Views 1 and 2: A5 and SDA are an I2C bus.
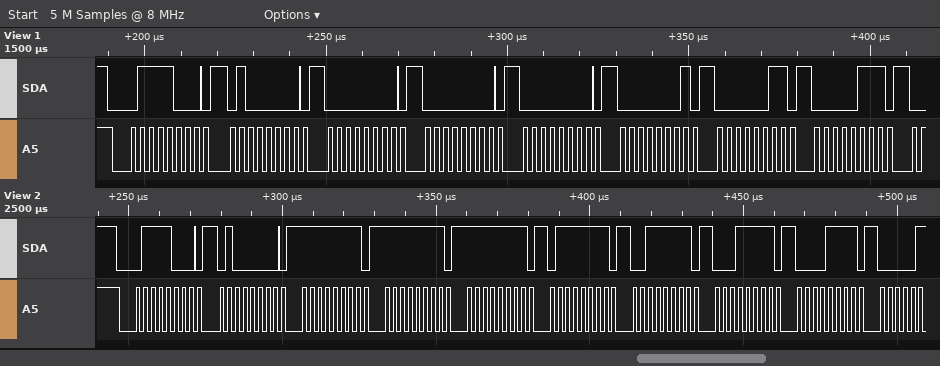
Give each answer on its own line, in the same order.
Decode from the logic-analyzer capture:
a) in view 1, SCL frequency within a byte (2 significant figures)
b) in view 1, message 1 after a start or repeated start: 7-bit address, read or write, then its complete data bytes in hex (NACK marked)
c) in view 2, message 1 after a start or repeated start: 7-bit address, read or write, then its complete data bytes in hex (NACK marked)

400 kHz
0x3C write: 40 00 00 00 01 03 07
0x3C write: 40 FF FF FF 7F 3F 1F 0F
